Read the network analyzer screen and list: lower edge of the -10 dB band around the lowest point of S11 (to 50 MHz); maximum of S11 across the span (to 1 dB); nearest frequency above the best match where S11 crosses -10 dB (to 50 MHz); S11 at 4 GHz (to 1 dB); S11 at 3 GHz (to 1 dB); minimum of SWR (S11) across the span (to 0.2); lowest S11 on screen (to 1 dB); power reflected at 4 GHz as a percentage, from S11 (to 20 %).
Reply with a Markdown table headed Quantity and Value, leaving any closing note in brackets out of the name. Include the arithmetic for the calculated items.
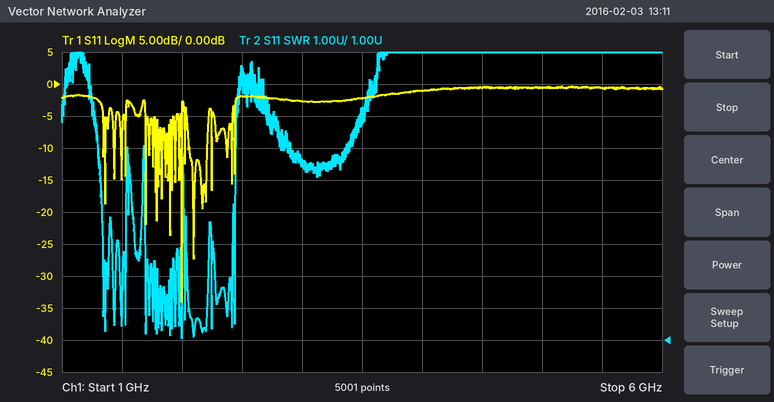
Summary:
| Quantity | Value |
|---|---|
| lower edge of the -10 dB band around the lowest point of S11 | 2.00 GHz |
| maximum of S11 across the span | 0 dB |
| nearest frequency above the best match where S11 crosses -10 dB | 2.00 GHz |
| S11 at 4 GHz | -1 dB |
| S11 at 3 GHz | -3 dB |
| minimum of SWR (S11) across the span | 1.0 |
| lowest S11 on screen | -34 dB |
| power reflected at 4 GHz as a percentage, from S11 | 10^(-1/10) ≈ 79.4 %, so 80 % to the nearest 20 % |
